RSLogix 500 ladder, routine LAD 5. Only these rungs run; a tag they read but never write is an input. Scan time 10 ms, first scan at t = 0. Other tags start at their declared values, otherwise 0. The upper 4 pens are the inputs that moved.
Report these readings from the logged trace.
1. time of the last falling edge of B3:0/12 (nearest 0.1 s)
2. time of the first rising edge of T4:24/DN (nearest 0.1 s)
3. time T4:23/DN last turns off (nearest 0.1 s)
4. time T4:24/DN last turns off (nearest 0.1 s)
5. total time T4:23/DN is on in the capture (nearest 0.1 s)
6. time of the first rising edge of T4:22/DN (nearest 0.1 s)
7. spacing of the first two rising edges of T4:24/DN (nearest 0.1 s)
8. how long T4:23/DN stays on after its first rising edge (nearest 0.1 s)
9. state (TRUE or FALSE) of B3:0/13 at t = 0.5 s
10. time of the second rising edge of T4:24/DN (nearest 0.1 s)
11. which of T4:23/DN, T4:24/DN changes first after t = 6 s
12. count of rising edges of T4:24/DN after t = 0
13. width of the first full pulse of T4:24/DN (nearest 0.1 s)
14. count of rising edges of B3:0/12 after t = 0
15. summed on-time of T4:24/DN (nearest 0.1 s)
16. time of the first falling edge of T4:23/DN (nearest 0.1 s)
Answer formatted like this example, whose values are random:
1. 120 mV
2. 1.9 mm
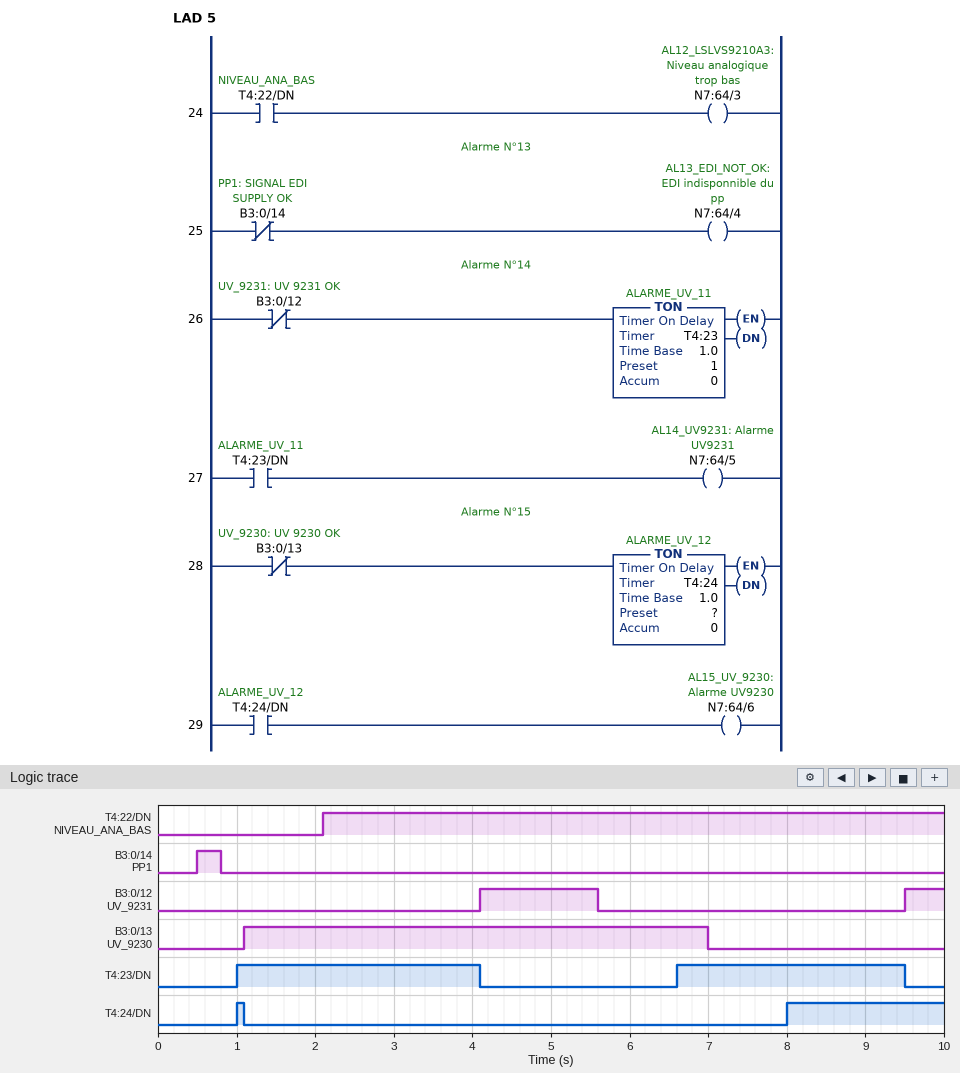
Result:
1. 5.6 s
2. 1.0 s
3. 9.5 s
4. 1.1 s
5. 6.0 s
6. 2.1 s
7. 7.0 s
8. 3.1 s
9. FALSE
10. 8.0 s
11. T4:23/DN
12. 2
13. 0.1 s
14. 2
15. 2.1 s
16. 4.1 s
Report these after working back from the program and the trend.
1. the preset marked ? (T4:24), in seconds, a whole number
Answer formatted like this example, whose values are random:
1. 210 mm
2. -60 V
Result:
1. 1 s
